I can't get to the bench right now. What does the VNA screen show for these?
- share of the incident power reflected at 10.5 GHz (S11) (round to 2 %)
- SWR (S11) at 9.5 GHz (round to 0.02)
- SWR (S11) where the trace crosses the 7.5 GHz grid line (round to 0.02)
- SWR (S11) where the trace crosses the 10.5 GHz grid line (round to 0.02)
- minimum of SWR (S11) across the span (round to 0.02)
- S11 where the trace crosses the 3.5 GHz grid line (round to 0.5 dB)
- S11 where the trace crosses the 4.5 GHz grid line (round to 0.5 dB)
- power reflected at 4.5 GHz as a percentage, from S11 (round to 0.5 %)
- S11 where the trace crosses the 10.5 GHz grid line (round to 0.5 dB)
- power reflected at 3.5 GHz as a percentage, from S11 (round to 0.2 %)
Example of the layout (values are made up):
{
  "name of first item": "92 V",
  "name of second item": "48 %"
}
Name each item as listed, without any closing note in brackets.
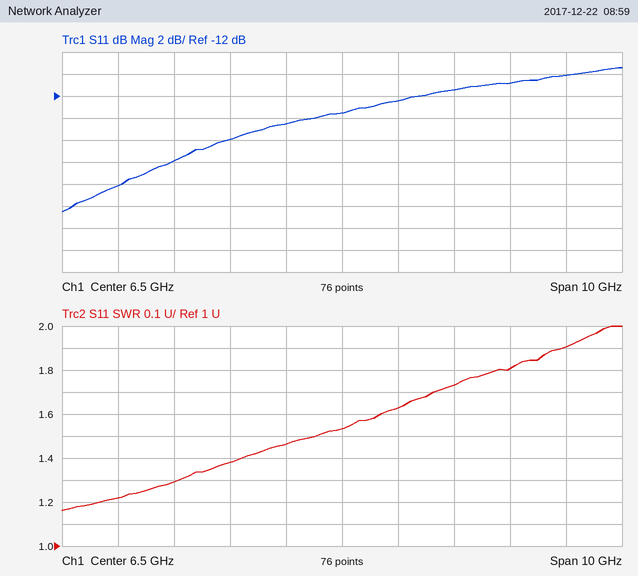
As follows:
{
  "share of the incident power reflected at 10.5 GHz (S11)": "10 %",
  "SWR (S11) at 9.5 GHz": "1.80",
  "SWR (S11) where the trace crosses the 7.5 GHz grid line": "1.62",
  "SWR (S11) where the trace crosses the 10.5 GHz grid line": "1.90",
  "minimum of SWR (S11) across the span": "1.16",
  "S11 where the trace crosses the 3.5 GHz grid line": "-18.0 dB",
  "S11 where the trace crosses the 4.5 GHz grid line": "-16.0 dB",
  "power reflected at 4.5 GHz as a percentage, from S11": "2.5 %",
  "S11 where the trace crosses the 10.5 GHz grid line": "-10.0 dB",
  "power reflected at 3.5 GHz as a percentage, from S11": "1.6 %"
}
